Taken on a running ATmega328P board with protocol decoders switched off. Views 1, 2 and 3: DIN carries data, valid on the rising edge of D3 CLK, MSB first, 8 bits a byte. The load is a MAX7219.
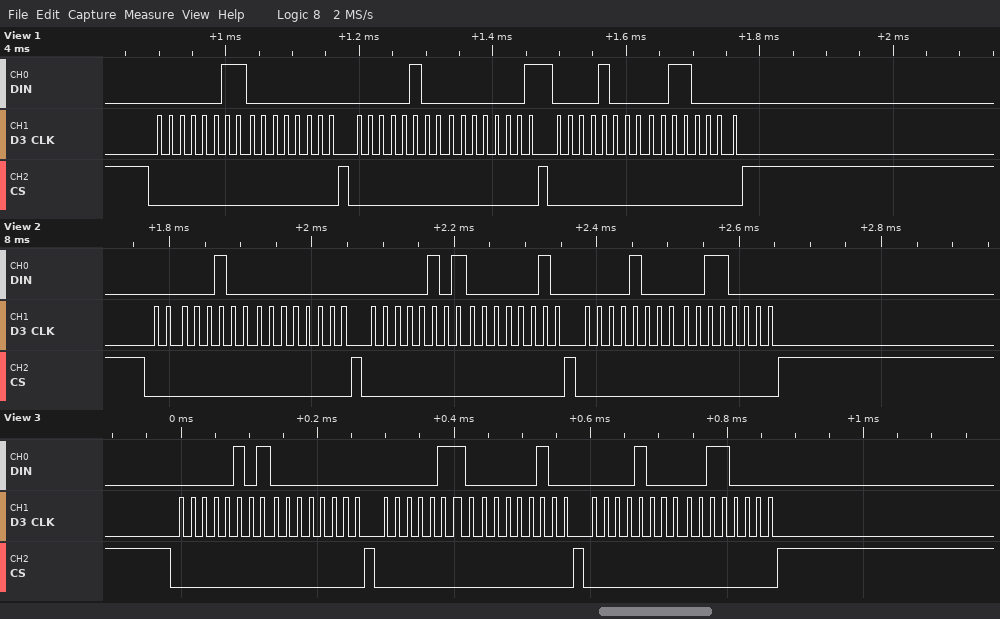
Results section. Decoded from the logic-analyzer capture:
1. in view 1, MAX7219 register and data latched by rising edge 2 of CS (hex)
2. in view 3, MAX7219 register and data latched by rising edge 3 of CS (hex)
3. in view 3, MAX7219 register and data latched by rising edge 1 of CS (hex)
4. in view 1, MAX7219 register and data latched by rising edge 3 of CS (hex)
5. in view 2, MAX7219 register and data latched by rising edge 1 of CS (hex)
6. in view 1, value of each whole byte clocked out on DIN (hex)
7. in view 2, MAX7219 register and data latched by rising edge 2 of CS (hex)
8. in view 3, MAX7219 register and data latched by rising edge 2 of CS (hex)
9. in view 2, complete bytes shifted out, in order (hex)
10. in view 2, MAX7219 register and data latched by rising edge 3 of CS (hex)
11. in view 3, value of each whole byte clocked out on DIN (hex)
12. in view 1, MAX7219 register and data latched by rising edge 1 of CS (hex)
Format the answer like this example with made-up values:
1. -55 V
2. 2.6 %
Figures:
1. register 0x4, data 0x01
2. register 0x8, data 0x30
3. register 0x5, data 0x00
4. register 0x8, data 0x30
5. register 0x4, data 0x00
6. 03 00 04 01 08 30
7. register 0x5, data 0x02
8. register 0x6, data 0x04
9. 04 00 05 02 08 30
10. register 0x8, data 0x30
11. 0x05 0x00 0x06 0x04 0x08 0x30
12. register 0x3, data 0x00
